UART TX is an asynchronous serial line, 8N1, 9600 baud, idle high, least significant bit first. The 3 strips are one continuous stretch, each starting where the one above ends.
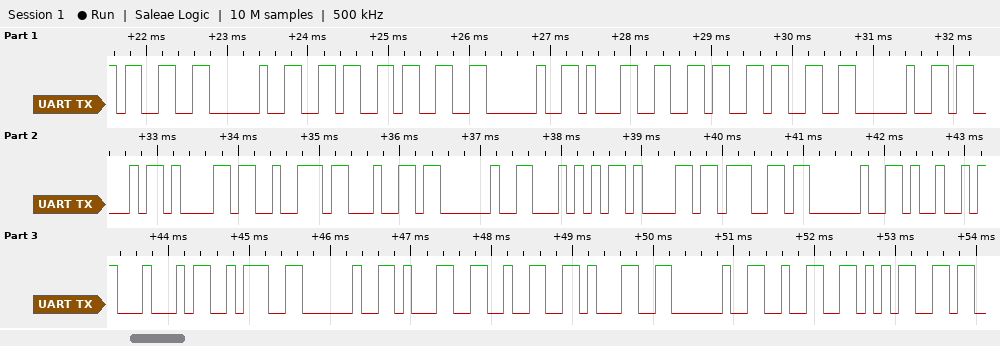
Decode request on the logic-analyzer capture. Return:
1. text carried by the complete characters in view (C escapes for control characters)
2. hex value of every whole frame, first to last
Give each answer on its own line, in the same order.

"3 63 163 Card Tag ID: 121 25"
33 20 36 33 20 31 36 33 20 43 61 72 64 20 54 61 67 20 49 44 3A 20 31 32 31 20 32 35
